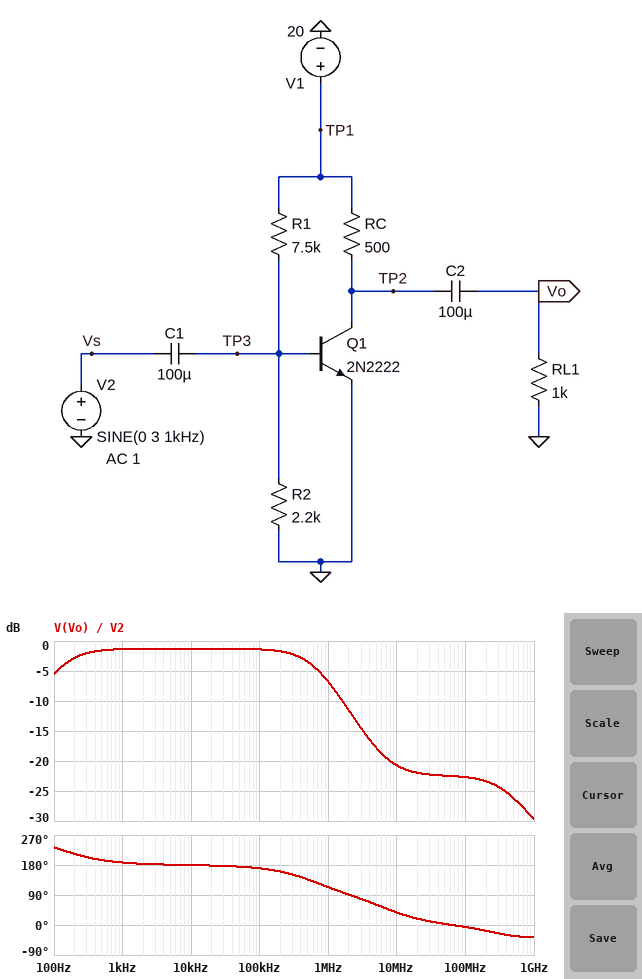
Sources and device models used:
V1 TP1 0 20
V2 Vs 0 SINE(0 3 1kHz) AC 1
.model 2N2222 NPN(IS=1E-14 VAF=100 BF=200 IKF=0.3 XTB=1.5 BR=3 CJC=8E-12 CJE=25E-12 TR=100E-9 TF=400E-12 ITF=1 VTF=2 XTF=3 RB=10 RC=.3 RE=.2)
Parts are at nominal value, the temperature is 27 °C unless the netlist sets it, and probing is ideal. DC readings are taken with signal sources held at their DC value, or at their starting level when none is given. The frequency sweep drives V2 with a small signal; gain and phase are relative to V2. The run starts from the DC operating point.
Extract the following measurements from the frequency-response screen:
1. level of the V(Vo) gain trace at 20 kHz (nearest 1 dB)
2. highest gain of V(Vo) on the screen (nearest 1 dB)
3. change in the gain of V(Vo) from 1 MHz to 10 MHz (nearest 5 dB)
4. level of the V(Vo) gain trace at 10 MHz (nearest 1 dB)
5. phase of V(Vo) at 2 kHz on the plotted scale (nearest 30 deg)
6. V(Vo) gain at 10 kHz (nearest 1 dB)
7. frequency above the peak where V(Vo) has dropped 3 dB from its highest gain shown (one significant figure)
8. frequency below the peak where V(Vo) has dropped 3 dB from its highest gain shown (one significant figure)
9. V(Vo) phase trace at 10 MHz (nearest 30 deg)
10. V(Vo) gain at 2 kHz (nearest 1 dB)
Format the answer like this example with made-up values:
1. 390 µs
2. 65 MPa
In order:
1. -1 dB
2. -1 dB
3. -15 dB
4. -21 dB
5. 180 deg
6. -1 dB
7. 600 kHz
8. 100 Hz
9. 30 deg
10. -1 dB
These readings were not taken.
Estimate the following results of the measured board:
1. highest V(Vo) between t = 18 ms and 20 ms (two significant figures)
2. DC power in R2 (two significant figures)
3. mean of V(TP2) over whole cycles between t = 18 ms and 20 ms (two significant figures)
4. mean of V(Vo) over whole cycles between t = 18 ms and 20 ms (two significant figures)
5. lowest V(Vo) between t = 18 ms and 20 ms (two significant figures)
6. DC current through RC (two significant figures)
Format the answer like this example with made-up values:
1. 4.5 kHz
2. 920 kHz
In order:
1. 12 V
2. 280 µW
3. 11 V
4. 9.6 V
5. -1.8 V
6. 40 mA
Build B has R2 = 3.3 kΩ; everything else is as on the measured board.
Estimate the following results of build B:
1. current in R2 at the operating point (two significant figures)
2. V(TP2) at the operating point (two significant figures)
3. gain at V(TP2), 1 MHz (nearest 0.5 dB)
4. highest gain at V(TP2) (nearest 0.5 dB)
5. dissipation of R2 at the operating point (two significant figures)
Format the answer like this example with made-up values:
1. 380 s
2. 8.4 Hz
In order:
1. 240 µA
2. 77 mV
3. -7.5 dB
4. -2.0 dB
5. 190 µW
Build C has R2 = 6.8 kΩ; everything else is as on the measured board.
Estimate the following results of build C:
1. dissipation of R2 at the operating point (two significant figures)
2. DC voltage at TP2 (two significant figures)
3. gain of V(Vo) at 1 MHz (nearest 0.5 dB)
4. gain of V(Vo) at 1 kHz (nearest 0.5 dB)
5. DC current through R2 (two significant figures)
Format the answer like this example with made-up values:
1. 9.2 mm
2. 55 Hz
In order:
1. 92 µW
2. 76 mV
3. -8.0 dB
4. -2.5 dB
5. 120 µA
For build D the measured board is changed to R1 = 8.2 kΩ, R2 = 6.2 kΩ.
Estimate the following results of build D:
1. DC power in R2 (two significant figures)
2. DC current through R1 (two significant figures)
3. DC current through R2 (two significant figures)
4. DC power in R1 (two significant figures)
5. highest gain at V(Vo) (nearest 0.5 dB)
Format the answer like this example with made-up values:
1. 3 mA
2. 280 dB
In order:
1. 100 µW
2. 2.3 mA
3. 130 µA
4. 45 mW
5. -1.5 dB
